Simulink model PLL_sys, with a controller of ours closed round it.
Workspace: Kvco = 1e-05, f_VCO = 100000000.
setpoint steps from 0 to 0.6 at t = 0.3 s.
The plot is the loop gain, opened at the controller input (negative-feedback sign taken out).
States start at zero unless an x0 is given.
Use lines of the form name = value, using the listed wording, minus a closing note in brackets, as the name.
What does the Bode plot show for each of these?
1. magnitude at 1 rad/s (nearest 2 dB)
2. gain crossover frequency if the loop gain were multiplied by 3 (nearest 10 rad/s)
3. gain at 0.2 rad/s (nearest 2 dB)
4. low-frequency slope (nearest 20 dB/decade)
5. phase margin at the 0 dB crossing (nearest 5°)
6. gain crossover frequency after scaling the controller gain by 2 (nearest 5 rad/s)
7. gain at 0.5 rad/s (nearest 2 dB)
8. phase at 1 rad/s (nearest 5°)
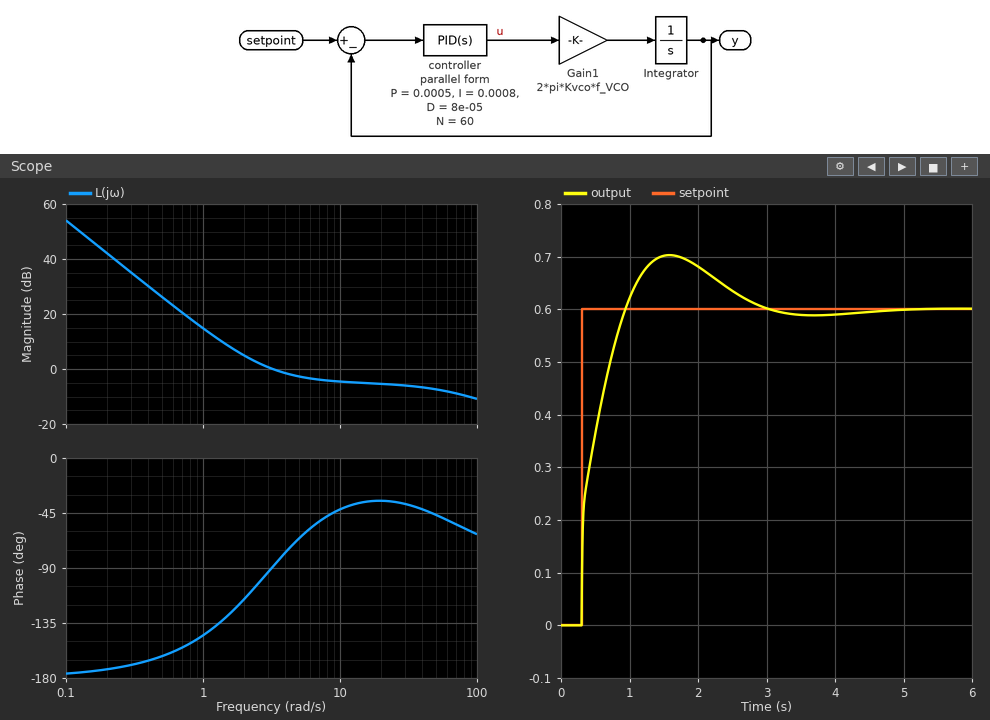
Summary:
magnitude at 1 rad/s = 14 dB
gain crossover frequency if the loop gain were multiplied by 3 = 80 rad/s
gain at 0.2 rad/s = 42 dB
low-frequency slope = -40 dB/decade
phase margin at the 0 dB crossing = 90°
gain crossover frequency after scaling the controller gain by 2 = 30 rad/s
gain at 0.5 rad/s = 26 dB
phase at 1 rad/s = -145°
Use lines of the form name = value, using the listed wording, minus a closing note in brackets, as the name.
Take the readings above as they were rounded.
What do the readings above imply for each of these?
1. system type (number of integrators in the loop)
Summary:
system type = 2
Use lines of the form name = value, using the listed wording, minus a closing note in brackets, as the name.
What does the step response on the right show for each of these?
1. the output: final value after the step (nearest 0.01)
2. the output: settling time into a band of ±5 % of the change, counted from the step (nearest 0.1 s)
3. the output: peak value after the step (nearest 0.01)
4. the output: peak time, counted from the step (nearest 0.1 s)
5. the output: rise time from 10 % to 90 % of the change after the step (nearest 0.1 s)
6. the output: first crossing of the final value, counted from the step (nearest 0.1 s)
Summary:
the output: final value after the step = 0.60
the output: settling time into a band of ±5 % of the change, counted from the step = 2.3 s
the output: peak value after the step = 0.70
the output: peak time, counted from the step = 1.3 s
the output: rise time from 10 % to 90 % of the change after the step = 0.5 s
the output: first crossing of the final value, counted from the step = 0.6 s
